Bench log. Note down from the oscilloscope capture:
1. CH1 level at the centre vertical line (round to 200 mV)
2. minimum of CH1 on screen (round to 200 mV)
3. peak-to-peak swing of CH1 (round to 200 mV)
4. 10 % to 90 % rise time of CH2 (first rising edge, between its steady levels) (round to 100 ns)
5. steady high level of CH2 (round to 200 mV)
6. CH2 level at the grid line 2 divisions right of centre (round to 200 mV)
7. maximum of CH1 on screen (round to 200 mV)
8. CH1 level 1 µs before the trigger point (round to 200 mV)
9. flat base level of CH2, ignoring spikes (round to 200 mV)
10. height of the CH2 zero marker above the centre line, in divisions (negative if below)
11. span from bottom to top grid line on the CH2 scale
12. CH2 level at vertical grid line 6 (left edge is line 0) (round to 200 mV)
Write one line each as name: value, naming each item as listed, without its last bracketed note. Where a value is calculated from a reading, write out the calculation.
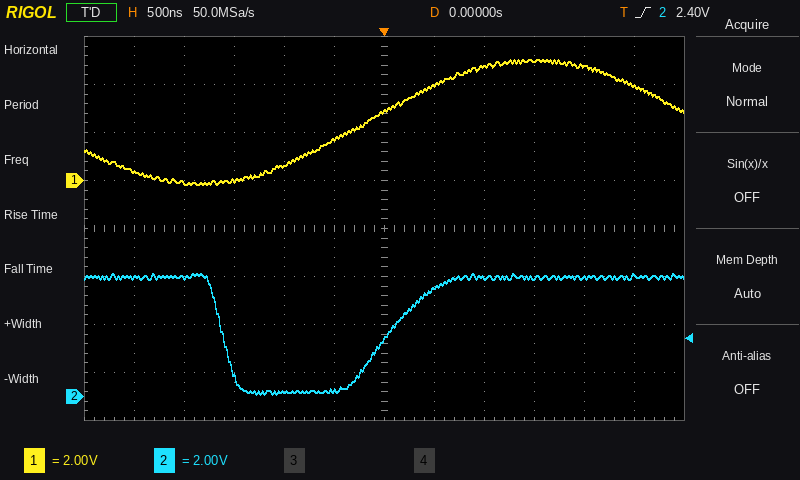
CH1 level at the centre vertical line: 2.8 V
minimum of CH1 on screen: -200 mV
peak-to-peak swing of CH1: 5.0 V − (-200 mV) = 5.2 V
10 % to 90 % rise time of CH2 (first rising edge, between its steady levels): 800 ns
steady high level of CH2: 5.0 V
CH2 level at the grid line 2 divisions right of centre: 5.0 V
maximum of CH1 on screen: 5.0 V
CH1 level 1 µs before the trigger point: 600 mV
flat base level of CH2, ignoring spikes: 200 mV
height of the CH2 zero marker above the centre line, in divisions: -3.5 div
span from bottom to top grid line on the CH2 scale: 16 V
CH2 level at vertical grid line 6 (left edge is line 0): 2.4 V
